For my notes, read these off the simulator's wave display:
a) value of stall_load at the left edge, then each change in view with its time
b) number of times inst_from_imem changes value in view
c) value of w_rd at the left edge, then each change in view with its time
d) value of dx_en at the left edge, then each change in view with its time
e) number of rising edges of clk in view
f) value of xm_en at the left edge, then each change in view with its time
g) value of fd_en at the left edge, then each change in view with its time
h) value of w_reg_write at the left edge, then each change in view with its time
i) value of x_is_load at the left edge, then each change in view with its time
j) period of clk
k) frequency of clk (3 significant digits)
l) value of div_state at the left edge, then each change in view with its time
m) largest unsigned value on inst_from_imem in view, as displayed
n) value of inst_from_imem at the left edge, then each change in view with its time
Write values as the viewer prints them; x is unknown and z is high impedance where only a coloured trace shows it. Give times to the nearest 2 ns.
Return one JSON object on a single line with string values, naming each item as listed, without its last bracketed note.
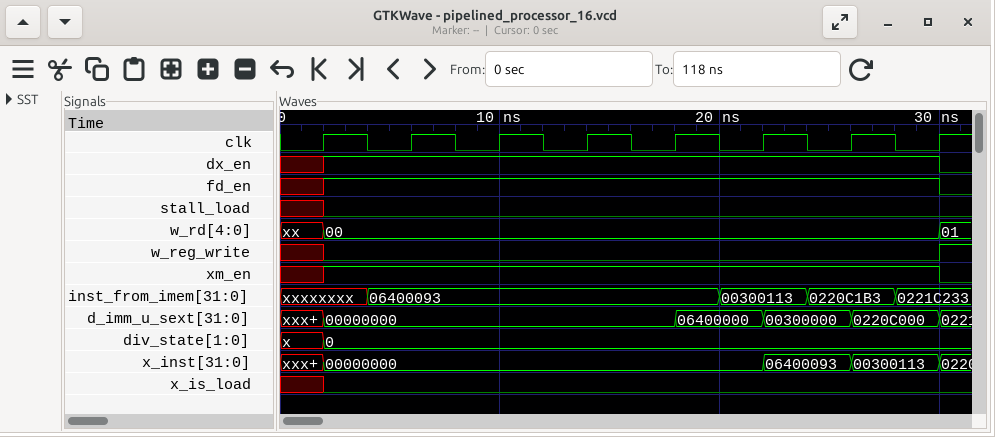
{"value of stall_load at the left edge, then each change in view with its time": "x, 0 at 2 ns", "number of times inst_from_imem changes value in view": "4", "value of w_rd at the left edge, then each change in view with its time": "xx, 00 at 2 ns, 01 at 30 ns", "value of dx_en at the left edge, then each change in view with its time": "x, 1 at 2 ns, 0 at 30 ns", "number of rising edges of clk in view": "8", "value of xm_en at the left edge, then each change in view with its time": "x, 1 at 2 ns, 0 at 30 ns", "value of fd_en at the left edge, then each change in view with its time": "x, 1 at 2 ns, 0 at 30 ns", "value of w_reg_write at the left edge, then each change in view with its time": "x, 0 at 2 ns, 1 at 30 ns", "value of x_is_load at the left edge, then each change in view with its time": "x, 0 at 2 ns", "period of clk": "4 ns", "frequency of clk": "250 MHz", "value of div_state at the left edge, then each change in view with its time": "x, 0 at 2 ns", "largest unsigned value on inst_from_imem in view, as displayed": "06400093", "value of inst_from_imem at the left edge, then each change in view with its time": "xxxxxxxx, 06400093 at 4 ns, 00300113 at 20 ns, 0220C1B3 at 24 ns, 0221C233 at 28 ns"}
